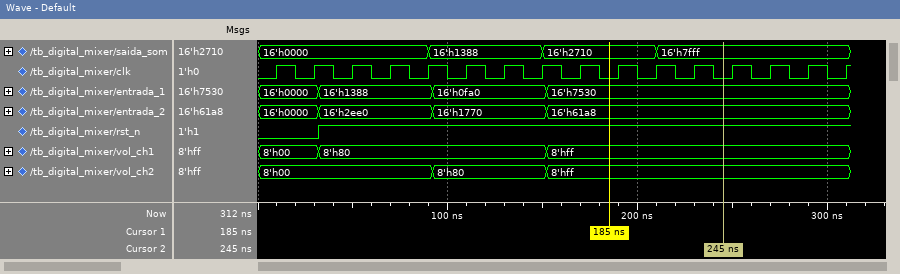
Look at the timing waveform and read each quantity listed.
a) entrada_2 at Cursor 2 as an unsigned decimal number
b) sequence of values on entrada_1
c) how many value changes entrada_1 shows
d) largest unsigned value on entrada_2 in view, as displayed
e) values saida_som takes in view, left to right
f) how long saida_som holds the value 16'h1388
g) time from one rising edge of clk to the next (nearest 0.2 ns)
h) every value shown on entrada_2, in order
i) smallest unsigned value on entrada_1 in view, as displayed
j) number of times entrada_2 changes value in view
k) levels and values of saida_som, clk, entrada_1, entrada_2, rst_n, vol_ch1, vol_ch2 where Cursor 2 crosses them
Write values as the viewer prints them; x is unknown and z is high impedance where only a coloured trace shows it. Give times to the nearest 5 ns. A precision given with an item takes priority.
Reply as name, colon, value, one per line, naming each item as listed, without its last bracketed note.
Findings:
entrada_2 at Cursor 2 as an unsigned decimal number: 25000
sequence of values on entrada_1: 16'h0000, 16'h1388, 16'h0fa0, 16'h7530
how many value changes entrada_1 shows: 3
largest unsigned value on entrada_2 in view, as displayed: 16'h61a8
values saida_som takes in view, left to right: 16'h0000, 16'h1388, 16'h2710, 16'h7fff
how long saida_som holds the value 16'h1388: 60 ns
time from one rising edge of clk to the next: 20 ns
every value shown on entrada_2, in order: 16'h0000, 16'h2ee0, 16'h1770, 16'h61a8
smallest unsigned value on entrada_1 in view, as displayed: 16'h0000
number of times entrada_2 changes value in view: 3
levels and values of saida_som, clk, entrada_1, entrada_2, rst_n, vol_ch1, vol_ch2 where Cursor 2 crosses them: saida_som=16'h7fff, clk=0, entrada_1=16'h7530, entrada_2=16'h61a8, rst_n=1, vol_ch1=8'hff, vol_ch2=8'hff
